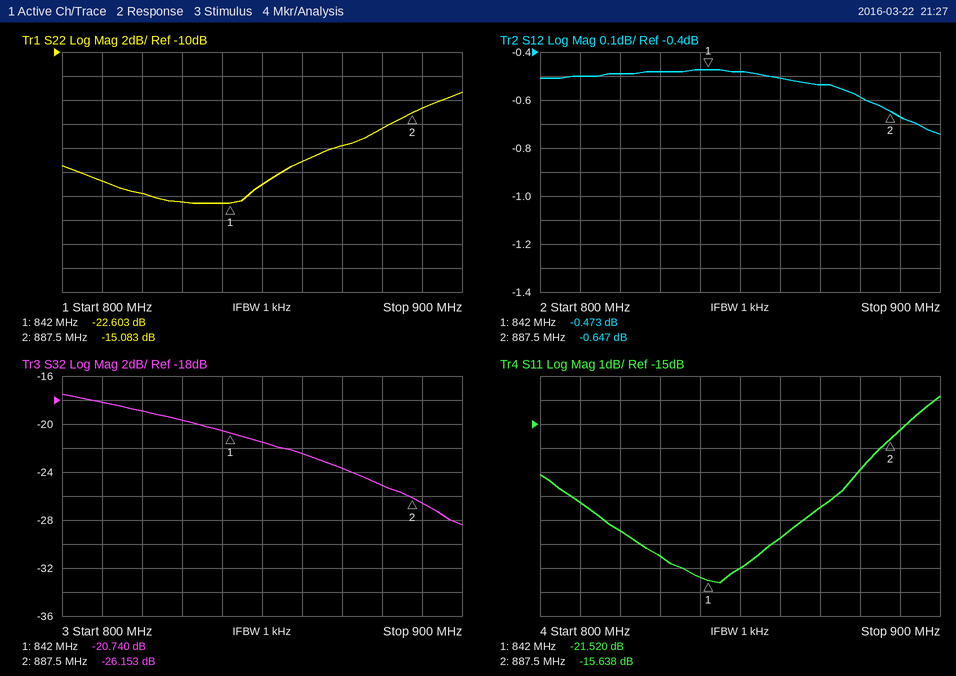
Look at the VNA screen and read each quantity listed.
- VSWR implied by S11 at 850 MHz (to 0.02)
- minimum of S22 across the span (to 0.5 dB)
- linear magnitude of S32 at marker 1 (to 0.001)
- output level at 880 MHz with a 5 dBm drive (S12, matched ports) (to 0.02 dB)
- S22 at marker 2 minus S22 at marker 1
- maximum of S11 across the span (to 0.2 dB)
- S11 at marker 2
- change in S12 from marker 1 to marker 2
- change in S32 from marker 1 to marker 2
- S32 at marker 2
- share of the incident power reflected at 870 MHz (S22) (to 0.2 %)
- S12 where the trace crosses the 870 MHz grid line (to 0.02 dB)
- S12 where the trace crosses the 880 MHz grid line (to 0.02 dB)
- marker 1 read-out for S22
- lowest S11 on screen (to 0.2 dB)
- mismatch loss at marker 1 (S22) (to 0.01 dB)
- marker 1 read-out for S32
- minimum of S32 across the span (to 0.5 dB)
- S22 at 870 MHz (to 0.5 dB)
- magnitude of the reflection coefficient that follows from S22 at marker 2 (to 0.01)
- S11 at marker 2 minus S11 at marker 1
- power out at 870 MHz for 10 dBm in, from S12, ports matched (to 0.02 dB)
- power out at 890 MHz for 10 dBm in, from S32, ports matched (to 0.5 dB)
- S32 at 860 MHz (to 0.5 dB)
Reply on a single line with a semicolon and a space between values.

1.20; -22.5 dB; 0.092; 4.42 dBm; 7.520 dB; -13.8 dB; -15.638 dB; -0.174 dB; -5.413 dB; -26.153 dB; 1.6 %; -0.54 dB; -0.58 dB; -22.603 dB; -21.6 dB; 0.02 dB; -20.740 dB; -28.5 dB; -18.0 dB; 0.18; 5.882 dB; 9.46 dBm; -16.5 dBm; -22.5 dB
